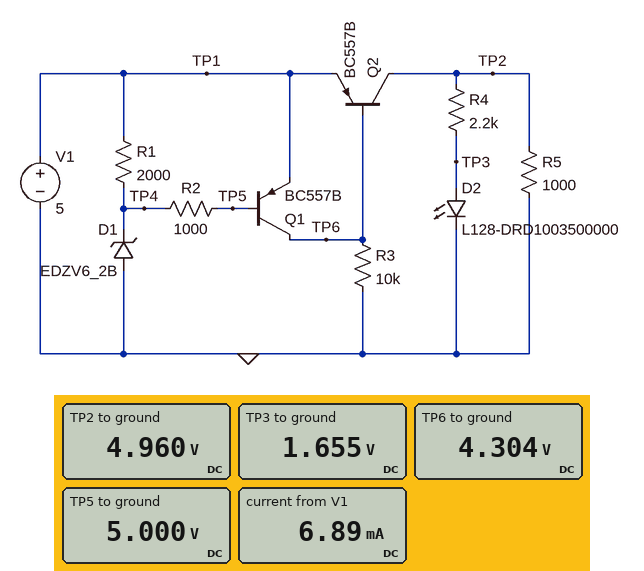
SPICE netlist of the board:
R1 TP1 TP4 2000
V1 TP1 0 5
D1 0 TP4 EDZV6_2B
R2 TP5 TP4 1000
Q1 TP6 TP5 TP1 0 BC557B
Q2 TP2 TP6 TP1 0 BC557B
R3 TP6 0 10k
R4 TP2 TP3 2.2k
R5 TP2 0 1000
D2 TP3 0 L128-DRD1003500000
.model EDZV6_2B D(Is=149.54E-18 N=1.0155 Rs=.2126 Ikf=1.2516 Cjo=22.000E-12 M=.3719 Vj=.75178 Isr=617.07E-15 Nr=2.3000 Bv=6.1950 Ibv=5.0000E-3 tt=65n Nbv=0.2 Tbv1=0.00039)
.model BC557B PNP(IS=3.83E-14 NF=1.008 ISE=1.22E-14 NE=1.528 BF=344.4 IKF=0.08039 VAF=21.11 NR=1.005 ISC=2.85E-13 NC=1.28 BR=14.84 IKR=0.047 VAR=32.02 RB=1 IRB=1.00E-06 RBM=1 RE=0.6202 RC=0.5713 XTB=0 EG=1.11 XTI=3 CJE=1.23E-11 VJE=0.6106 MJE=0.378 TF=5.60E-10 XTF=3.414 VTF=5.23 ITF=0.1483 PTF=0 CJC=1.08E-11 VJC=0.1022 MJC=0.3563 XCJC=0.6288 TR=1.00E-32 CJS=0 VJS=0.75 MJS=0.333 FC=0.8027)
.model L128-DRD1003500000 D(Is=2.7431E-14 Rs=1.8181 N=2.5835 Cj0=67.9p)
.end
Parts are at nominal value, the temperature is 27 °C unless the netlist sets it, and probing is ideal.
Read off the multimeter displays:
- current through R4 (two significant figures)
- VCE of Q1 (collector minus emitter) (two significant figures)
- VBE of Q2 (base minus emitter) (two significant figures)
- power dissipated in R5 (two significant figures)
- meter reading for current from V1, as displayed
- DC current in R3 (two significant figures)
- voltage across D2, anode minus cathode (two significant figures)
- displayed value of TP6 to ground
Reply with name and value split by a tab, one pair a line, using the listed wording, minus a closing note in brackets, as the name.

current through R4	1.5 mA
VCE of Q1 (collector minus emitter)	-700 mV
VBE of Q2 (base minus emitter)	-700 mV
power dissipated in R5	25 mW
meter reading for current from V1, as displayed	6.89 mA
DC current in R3	430 µA
voltage across D2, anode minus cathode	1.7 V
displayed value of TP6 to ground	4.304 V
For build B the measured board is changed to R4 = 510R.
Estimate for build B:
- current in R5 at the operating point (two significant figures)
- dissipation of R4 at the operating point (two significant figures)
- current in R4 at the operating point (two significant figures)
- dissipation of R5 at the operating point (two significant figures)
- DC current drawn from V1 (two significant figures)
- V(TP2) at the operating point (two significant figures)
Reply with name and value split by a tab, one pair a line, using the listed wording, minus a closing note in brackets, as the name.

current in R5 at the operating point	4.9 mA
dissipation of R4 at the operating point	20 mW
current in R4 at the operating point	6.2 mA
dissipation of R5 at the operating point	24 mW
DC current drawn from V1	12 mA
V(TP2) at the operating point	4.9 V
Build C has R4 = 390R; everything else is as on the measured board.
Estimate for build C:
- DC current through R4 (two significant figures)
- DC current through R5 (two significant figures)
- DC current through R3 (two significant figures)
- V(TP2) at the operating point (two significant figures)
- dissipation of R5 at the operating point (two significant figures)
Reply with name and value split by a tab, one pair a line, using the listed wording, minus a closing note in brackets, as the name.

DC current through R4	8.1 mA
DC current through R5	4.9 mA
DC current through R3	430 µA
V(TP2) at the operating point	4.9 V
dissipation of R5 at the operating point	24 mW
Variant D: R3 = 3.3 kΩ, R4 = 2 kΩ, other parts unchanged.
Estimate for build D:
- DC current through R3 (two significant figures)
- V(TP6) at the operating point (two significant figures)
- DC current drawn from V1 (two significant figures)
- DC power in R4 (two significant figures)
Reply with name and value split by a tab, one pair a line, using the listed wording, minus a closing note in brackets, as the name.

DC current through R3	1.3 mA
V(TP6) at the operating point	4.3 V
DC current drawn from V1	7.9 mA
DC power in R4	5.5 mW
